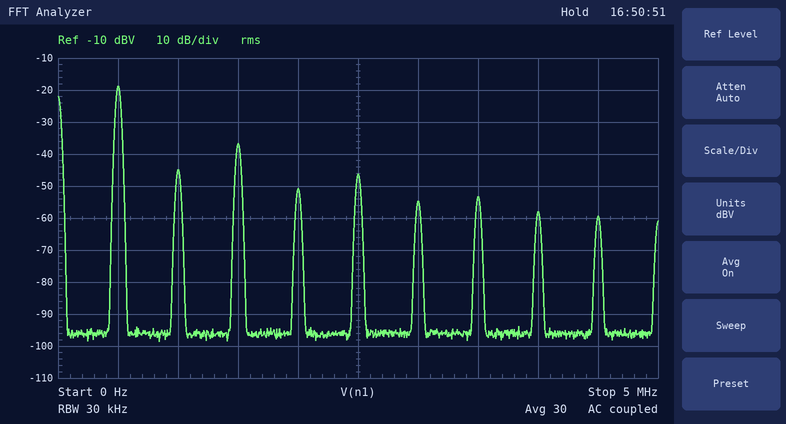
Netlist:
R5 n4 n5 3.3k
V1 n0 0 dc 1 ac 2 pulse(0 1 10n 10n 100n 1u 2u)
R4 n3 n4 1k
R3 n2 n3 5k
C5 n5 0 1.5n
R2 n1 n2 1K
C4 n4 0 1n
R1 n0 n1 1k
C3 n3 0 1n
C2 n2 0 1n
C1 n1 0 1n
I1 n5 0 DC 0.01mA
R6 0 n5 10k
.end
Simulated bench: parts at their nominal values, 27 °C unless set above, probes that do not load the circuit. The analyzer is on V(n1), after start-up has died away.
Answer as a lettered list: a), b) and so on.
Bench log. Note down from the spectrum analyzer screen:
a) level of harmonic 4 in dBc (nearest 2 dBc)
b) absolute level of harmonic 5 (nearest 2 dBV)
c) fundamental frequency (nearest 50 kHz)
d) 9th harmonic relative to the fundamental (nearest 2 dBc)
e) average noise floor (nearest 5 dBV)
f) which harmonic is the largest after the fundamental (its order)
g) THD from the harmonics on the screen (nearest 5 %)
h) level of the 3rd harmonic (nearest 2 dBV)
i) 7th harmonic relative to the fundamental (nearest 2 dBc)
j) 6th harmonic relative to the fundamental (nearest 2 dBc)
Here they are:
a) -32 dBc
b) -46 dBV
c) 500 kHz
d) -40 dBc
e) -95 dBV
f) 3
g) 15 %
h) -36 dBV
i) -34 dBc
j) -36 dBc
